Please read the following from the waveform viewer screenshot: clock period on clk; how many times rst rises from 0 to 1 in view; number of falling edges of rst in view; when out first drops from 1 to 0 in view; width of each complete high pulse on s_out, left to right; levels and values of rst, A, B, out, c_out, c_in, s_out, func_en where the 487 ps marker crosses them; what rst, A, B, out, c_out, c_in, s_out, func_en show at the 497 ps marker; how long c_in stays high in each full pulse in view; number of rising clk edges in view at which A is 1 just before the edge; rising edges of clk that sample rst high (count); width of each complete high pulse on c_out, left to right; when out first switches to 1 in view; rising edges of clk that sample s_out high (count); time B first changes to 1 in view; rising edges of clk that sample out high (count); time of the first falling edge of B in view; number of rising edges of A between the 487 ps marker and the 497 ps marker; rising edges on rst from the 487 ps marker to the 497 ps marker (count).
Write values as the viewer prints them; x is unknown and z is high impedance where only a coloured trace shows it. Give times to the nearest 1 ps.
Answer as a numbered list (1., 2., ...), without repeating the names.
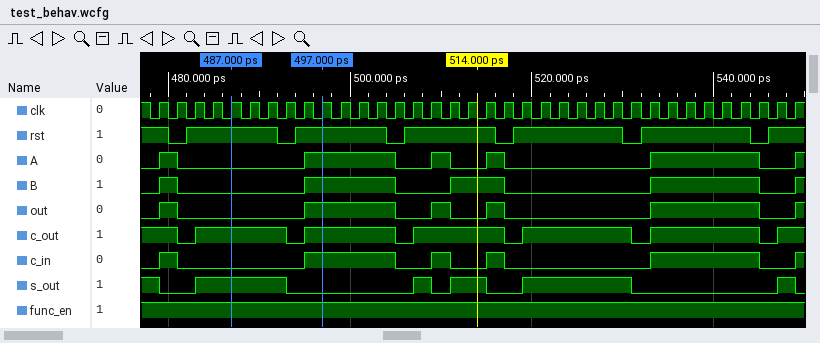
1. 2 ps
2. 6
3. 6
4. 481 ps
5. 10 ps, 2 ps, 4 ps, 12 ps, 2 ps
6. rst=1, A=0, B=0, out=0, c_out=1, c_in=0, s_out=1, func_en=1
7. rst=1, A=1, B=1, out=1, c_out=1, c_in=1, s_out=0, func_en=1
8. 2 ps, 10 ps, 2 ps, 2 ps, 12 ps
9. 14
10. 30
11. 10 ps, 10 ps, 10 ps, 12 ps, 12 ps
12. 479 ps
13. 16
14. 479 ps
15. 14
16. 481 ps
17. 1
18. 1
